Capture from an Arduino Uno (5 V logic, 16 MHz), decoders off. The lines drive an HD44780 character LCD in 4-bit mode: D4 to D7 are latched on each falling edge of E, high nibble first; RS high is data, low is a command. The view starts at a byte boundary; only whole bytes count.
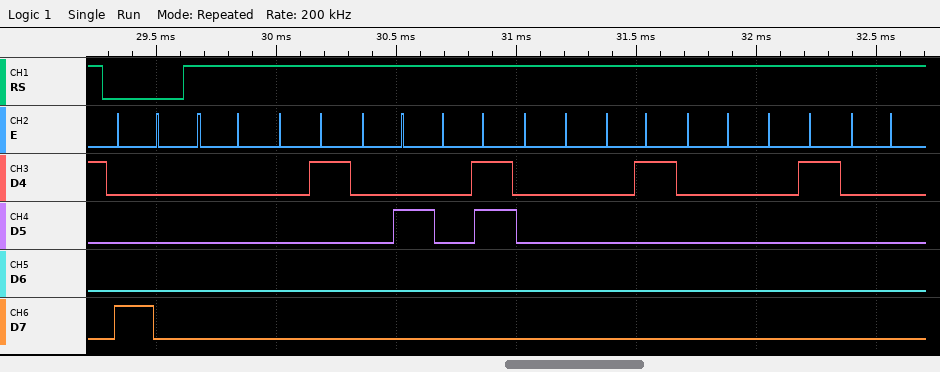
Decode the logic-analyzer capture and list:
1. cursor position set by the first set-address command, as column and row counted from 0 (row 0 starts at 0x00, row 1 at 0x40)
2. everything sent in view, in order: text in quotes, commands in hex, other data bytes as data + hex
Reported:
column 0, row 0
0x80 data 00 01 02 03 00 01 00 01 00
